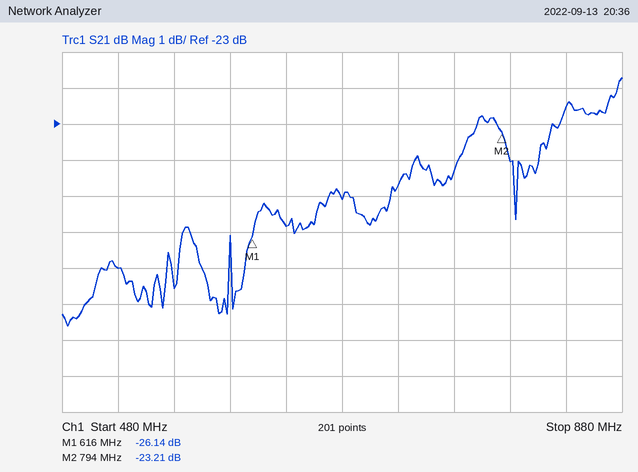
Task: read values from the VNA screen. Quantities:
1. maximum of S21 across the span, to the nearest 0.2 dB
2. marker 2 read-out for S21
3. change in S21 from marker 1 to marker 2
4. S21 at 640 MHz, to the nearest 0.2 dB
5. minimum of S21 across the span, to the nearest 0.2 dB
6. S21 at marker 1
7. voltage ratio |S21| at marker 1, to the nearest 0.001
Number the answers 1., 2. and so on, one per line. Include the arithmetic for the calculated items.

1. -21.8 dB
2. -23.21 dB
3. -23.21 − (-26.14) = 2.93 dB
4. -25.8 dB
5. -28.6 dB
6. -26.14 dB
7. 10^(-26.14/20) ≈ 0.049
